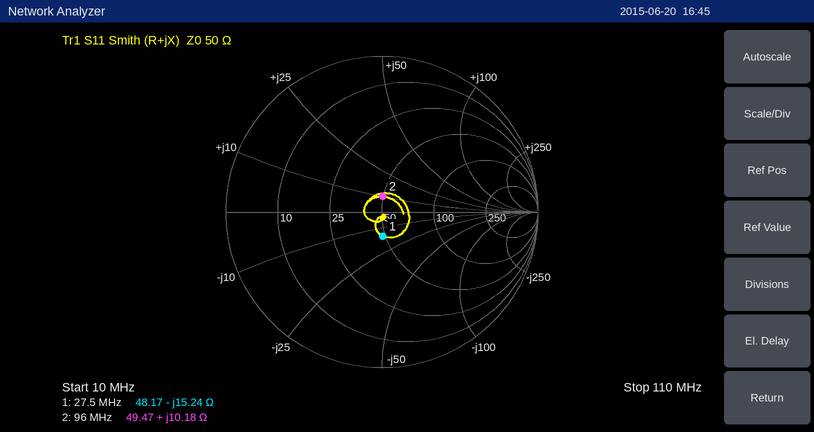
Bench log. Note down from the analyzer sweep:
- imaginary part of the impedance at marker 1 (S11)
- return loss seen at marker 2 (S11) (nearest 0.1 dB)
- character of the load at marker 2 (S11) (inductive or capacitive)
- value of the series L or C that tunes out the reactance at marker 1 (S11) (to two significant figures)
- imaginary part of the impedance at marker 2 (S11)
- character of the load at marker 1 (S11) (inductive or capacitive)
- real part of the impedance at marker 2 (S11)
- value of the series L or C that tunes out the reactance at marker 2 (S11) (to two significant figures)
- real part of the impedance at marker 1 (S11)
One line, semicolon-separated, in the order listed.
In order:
-15.24 Ω; 19.8 dB; inductive; 88 nH; +10.18 Ω; capacitive; 49.47 Ω; 160 pF; 48.17 Ω
